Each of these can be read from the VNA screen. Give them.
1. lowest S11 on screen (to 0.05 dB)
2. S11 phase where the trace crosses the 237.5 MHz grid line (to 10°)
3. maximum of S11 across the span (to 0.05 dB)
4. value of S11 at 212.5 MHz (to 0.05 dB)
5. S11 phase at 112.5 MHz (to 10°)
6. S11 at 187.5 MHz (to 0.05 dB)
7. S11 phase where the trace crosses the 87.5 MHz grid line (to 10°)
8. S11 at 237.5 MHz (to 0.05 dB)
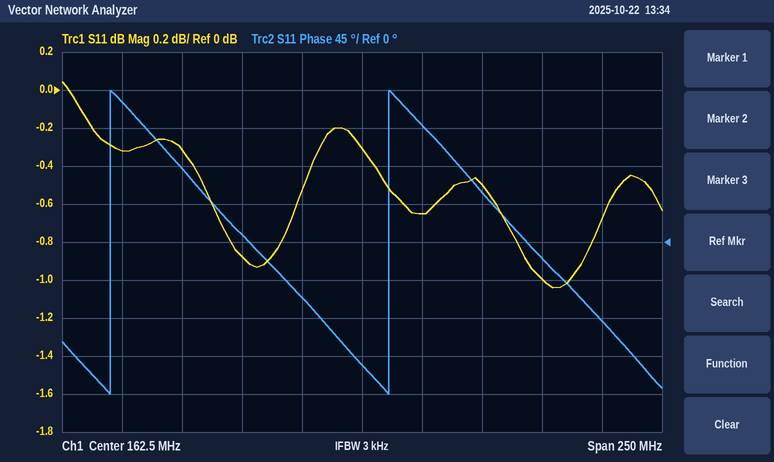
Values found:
-1.05 dB
-20°
0.05 dB
-0.50 dB
10°
-0.65 dB
90°
-1.00 dB
